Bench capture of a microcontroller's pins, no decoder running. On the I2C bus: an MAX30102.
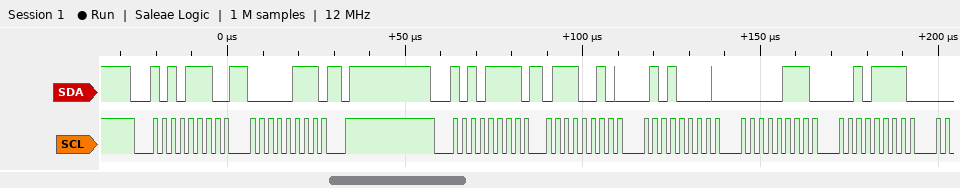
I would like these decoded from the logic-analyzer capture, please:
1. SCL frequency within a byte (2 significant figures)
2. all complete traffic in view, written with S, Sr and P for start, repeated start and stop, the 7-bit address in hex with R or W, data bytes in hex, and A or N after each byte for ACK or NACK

400 kHz
S 57W A 07 A P S 57R A 72 A 50 A 07 A 2F A
